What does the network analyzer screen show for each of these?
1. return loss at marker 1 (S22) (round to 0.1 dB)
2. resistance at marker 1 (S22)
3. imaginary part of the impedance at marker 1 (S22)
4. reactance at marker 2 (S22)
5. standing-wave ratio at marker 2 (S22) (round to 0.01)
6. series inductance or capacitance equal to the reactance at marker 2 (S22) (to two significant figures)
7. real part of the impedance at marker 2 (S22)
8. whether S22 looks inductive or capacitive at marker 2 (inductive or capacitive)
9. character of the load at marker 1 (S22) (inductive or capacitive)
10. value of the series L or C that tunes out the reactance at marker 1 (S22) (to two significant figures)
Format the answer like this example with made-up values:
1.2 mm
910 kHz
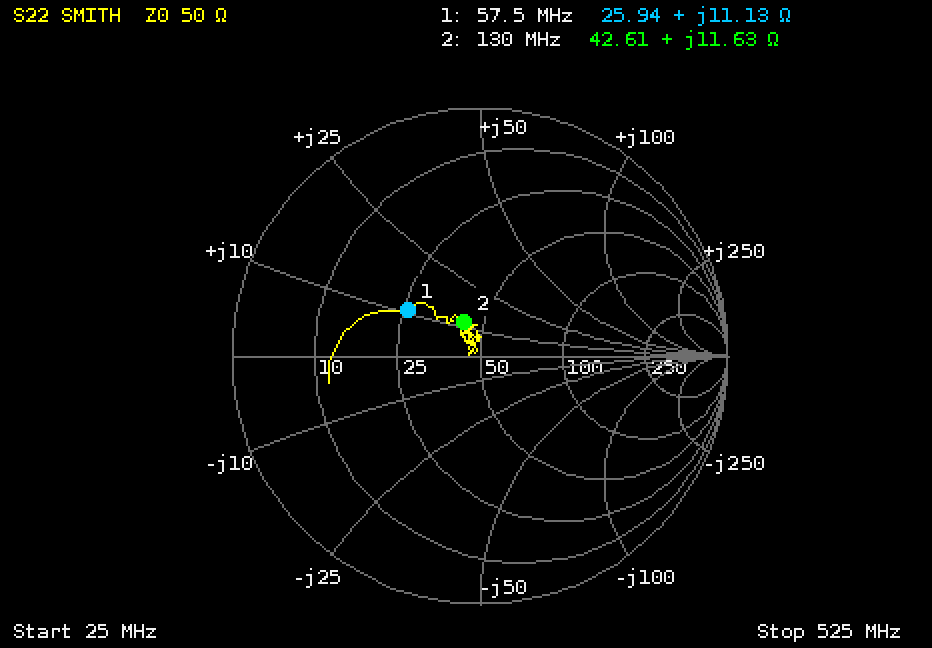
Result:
9.2 dB
25.94 Ω
+11.13 Ω
+11.63 Ω
1.35
14 nH
42.61 Ω
inductive
inductive
250 pF
